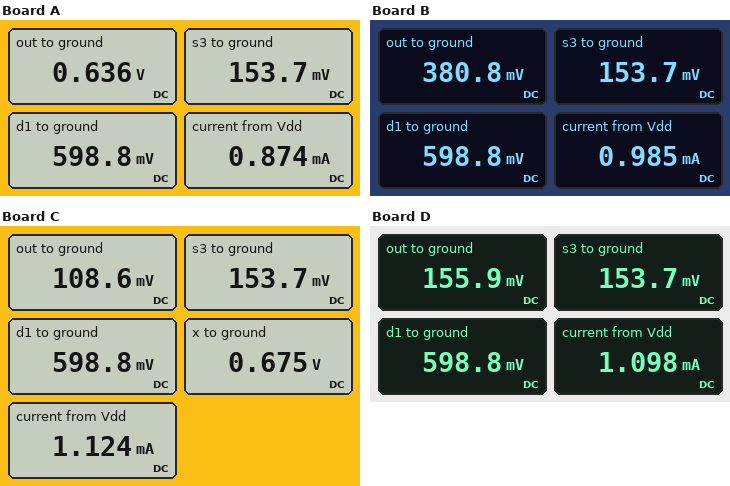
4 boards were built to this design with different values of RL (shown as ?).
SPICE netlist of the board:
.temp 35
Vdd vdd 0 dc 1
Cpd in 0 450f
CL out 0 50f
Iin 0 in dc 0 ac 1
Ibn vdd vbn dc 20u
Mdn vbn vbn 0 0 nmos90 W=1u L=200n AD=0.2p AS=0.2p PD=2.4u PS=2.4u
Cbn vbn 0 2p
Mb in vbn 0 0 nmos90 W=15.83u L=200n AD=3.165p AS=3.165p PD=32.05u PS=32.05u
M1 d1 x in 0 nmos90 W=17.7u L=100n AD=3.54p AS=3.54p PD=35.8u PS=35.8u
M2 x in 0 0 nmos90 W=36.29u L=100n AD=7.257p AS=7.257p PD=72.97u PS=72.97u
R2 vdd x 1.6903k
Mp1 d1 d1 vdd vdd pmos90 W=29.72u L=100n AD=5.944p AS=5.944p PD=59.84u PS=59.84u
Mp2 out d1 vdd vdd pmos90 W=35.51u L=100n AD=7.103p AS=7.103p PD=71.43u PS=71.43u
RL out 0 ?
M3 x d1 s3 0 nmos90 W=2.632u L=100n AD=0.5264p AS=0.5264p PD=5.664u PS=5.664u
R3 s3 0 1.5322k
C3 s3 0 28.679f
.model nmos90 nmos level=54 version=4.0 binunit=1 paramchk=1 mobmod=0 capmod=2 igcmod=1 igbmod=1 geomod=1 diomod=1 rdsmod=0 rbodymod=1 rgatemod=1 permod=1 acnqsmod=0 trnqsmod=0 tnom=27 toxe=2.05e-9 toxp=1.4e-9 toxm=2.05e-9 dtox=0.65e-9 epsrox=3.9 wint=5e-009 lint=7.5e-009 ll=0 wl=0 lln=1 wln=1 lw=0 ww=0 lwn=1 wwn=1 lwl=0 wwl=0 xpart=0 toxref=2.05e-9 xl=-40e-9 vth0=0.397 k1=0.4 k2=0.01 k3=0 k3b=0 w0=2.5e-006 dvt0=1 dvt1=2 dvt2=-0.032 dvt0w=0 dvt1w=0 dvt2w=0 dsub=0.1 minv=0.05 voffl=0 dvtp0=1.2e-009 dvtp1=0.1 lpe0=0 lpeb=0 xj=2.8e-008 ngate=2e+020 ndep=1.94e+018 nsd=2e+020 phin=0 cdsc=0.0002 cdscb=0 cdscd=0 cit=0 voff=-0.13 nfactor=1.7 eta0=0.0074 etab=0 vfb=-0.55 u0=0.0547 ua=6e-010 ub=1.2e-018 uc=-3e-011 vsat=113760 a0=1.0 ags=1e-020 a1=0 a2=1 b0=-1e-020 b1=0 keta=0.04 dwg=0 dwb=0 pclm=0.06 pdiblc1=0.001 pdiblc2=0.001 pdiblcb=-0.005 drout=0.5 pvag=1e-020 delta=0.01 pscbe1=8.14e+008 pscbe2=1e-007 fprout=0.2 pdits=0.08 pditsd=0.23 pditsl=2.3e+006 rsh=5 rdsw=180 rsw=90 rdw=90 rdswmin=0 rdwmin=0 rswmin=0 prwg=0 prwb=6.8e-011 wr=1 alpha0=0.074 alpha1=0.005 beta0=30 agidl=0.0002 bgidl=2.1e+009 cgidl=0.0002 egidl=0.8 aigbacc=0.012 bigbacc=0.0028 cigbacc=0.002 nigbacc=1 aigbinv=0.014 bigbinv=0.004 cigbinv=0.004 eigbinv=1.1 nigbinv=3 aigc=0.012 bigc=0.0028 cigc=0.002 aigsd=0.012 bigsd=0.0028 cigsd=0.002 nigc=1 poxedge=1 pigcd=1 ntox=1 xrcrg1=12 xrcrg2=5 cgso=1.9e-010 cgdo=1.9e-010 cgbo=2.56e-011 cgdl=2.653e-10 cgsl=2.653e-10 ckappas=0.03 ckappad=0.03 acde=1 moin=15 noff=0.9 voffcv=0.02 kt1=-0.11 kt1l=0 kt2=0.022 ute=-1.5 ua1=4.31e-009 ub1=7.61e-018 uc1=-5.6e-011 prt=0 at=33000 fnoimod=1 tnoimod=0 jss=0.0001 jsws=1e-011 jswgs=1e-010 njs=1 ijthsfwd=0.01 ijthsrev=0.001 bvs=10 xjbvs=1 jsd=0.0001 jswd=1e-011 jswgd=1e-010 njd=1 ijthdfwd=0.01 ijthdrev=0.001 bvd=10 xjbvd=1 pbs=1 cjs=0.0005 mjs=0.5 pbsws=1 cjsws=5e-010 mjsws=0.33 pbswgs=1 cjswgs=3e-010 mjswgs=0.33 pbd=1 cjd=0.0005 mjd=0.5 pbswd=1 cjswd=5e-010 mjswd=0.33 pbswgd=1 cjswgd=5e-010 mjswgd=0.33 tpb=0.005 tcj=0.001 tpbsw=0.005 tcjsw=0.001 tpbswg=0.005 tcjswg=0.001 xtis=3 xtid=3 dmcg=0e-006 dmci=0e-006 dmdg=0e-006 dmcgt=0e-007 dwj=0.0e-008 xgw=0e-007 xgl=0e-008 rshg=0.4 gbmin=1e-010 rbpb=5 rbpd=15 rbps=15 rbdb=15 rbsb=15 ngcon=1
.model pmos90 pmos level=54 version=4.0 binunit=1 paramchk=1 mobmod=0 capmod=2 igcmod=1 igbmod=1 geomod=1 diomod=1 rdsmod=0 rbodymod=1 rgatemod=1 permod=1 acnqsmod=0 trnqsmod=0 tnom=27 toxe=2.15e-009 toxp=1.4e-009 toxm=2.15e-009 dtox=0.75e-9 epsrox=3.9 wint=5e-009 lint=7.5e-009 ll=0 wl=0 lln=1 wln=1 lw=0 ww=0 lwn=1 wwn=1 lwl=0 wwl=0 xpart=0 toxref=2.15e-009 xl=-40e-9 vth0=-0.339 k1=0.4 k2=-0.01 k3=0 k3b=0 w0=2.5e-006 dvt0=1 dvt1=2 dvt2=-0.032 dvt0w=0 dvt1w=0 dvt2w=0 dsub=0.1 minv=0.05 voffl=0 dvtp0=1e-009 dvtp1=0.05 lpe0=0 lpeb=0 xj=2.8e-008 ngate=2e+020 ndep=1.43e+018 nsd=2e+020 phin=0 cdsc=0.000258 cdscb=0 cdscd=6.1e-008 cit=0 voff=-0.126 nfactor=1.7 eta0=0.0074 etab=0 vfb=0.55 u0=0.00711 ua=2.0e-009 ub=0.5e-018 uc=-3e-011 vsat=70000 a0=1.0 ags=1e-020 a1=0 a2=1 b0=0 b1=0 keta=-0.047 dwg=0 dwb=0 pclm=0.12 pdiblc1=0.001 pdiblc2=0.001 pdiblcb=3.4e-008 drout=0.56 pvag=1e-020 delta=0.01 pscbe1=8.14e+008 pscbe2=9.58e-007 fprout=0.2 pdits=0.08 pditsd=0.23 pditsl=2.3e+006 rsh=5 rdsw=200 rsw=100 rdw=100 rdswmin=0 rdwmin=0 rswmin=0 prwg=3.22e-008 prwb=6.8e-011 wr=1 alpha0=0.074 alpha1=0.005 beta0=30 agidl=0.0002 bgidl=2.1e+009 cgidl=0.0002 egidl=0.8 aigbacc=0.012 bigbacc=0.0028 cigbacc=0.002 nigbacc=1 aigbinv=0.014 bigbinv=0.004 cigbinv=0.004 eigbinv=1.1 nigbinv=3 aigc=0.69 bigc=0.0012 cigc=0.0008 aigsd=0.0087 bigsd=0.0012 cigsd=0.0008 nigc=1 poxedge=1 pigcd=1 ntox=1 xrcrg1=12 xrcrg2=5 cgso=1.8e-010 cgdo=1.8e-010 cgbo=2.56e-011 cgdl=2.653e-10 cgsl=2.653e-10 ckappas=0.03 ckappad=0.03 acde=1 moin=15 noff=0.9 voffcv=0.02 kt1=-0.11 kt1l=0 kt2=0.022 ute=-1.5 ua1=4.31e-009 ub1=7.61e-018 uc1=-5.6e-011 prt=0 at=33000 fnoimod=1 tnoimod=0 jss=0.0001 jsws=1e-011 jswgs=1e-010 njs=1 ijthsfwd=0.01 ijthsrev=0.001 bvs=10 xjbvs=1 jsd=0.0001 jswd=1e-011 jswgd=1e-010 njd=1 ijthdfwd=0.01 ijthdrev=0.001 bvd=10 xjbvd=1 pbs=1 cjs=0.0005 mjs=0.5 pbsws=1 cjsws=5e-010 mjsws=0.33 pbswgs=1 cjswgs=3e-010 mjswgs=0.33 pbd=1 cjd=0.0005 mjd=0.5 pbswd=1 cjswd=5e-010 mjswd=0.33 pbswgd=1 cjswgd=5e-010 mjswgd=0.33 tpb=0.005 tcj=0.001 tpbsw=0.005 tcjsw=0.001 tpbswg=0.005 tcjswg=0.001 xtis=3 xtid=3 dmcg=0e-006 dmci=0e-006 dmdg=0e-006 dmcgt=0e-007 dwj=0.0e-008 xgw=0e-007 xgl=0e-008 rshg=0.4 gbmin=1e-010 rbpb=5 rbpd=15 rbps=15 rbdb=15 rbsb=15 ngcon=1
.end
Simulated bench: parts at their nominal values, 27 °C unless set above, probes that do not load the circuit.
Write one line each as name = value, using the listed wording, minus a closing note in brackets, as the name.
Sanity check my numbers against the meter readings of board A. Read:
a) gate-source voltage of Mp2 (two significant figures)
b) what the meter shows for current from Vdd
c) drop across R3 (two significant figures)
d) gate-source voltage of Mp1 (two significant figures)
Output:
gate-source voltage of Mp2 = -400 mV
what the meter shows for current from Vdd = 0.874 mA
drop across R3 = 150 mV
gate-source voltage of Mp1 = -400 mV
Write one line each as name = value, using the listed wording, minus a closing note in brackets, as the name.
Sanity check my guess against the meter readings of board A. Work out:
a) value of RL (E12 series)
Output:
value of RL = 1.8 kΩ
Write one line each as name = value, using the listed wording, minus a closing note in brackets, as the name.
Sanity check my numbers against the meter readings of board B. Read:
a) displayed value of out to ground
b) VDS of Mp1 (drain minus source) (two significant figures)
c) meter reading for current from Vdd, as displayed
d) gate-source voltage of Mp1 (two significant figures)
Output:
displayed value of out to ground = 380.8 mV
VDS of Mp1 (drain minus source) = -400 mV
meter reading for current from Vdd, as displayed = 0.985 mA
gate-source voltage of Mp1 = -400 mV
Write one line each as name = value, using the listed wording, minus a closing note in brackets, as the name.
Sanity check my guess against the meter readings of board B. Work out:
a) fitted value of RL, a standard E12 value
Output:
fitted value of RL, a standard E12 value = 820 Ω
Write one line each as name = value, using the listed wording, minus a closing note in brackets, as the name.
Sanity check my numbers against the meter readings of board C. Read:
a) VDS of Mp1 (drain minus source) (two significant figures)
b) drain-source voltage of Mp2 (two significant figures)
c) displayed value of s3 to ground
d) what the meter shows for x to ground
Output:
VDS of Mp1 (drain minus source) = -400 mV
drain-source voltage of Mp2 = -890 mV
displayed value of s3 to ground = 153.7 mV
what the meter shows for x to ground = 0.675 V
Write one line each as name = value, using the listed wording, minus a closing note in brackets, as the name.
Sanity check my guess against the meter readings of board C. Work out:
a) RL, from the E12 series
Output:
RL, from the E12 series = 180 Ω
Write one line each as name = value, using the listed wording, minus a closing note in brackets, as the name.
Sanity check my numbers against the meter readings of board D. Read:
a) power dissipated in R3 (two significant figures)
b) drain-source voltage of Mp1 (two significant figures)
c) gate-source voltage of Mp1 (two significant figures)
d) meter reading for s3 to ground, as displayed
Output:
power dissipated in R3 = 15 µW
drain-source voltage of Mp1 = -400 mV
gate-source voltage of Mp1 = -400 mV
meter reading for s3 to ground, as displayed = 153.7 mV
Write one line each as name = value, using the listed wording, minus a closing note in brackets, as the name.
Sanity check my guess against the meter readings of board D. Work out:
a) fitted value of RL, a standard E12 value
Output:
fitted value of RL, a standard E12 value = 270 Ω
